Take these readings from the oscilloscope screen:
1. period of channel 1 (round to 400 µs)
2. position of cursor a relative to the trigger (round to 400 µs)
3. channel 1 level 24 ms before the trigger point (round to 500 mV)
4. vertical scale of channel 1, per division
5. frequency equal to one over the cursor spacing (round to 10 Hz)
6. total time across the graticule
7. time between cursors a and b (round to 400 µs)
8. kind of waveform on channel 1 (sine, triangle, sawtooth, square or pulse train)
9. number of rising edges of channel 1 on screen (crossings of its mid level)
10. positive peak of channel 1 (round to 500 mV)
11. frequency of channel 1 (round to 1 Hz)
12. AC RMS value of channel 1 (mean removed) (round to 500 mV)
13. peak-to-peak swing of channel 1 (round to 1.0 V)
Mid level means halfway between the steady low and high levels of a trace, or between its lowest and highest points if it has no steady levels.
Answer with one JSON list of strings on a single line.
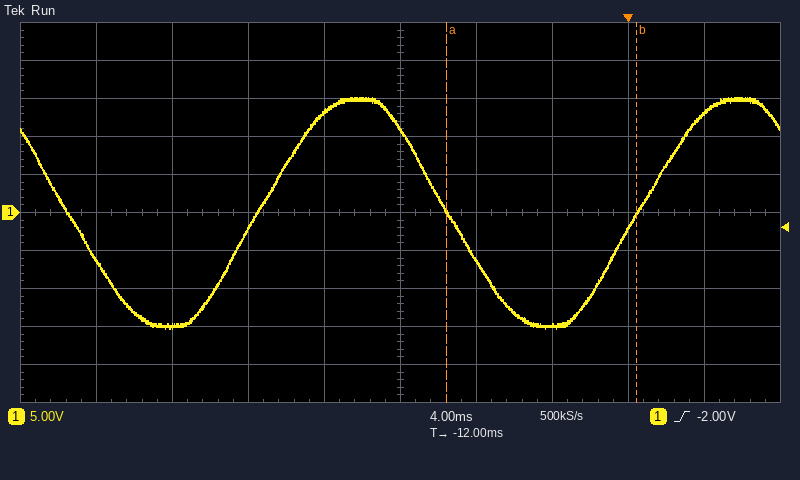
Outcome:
["20.0 ms", "-9.6 ms", "-15.0 V", "5 V", "100 Hz", "40 ms", "10.0 ms", "sine", "2", "15.0 V", "50 Hz", "10.5 V", "30.0 V"]
